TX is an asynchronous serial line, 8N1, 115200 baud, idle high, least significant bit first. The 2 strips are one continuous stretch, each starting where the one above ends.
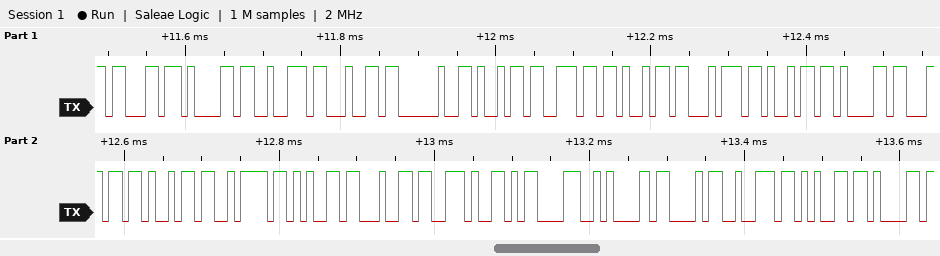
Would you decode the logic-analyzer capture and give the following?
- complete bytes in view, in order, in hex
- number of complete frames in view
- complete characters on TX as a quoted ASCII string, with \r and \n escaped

0x63 0x61 0x72 0x64 0x20 0x69 0x6E 0x69 0x74 0x69 0x61 0x6C 0x69 0x7A 0x65 0x64 0x2E 0x0D 0x0A 0x43 0x72 0x65 0x61
23
"card initialized.\r\nCrea"
